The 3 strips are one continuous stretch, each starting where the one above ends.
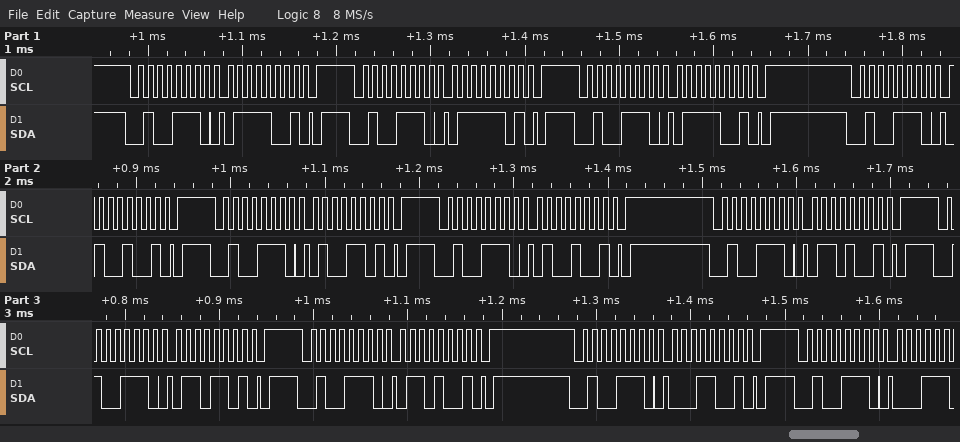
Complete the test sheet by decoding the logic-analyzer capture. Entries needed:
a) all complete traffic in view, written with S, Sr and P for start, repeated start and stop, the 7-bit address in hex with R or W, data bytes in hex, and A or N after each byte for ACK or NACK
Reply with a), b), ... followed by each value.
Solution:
a) S 27W A 79 A P S 27W A 7D A P S 27W A 79 A P S 27W A 49 A P S 27W A 4D A P S 27W A 49 A P S 27W A 69 A P S 27W A 6D A P S 27W A 69 A P S 27W A 19 A P S 27W A
